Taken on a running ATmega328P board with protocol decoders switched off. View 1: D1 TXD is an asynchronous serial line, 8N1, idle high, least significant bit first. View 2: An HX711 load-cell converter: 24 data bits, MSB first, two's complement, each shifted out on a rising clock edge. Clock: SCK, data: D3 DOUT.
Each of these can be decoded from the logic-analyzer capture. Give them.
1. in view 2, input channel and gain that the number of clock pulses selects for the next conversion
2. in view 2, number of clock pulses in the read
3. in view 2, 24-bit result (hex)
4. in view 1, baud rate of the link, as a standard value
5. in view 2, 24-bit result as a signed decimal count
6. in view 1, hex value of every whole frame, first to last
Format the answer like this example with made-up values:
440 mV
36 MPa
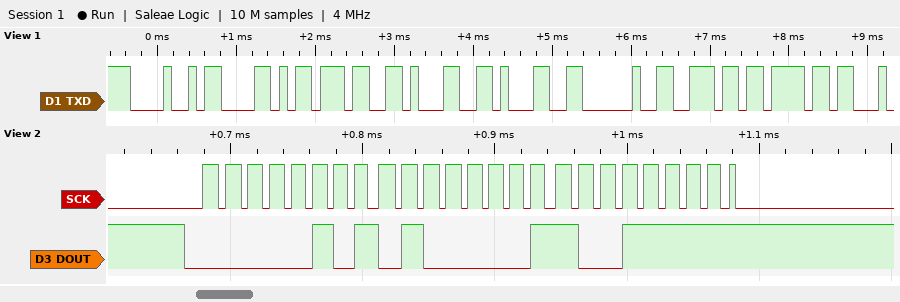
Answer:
channel A, gain 128
25
0x05419F
9600 baud
344479
48 58 37 31 31 20 6E 6F
